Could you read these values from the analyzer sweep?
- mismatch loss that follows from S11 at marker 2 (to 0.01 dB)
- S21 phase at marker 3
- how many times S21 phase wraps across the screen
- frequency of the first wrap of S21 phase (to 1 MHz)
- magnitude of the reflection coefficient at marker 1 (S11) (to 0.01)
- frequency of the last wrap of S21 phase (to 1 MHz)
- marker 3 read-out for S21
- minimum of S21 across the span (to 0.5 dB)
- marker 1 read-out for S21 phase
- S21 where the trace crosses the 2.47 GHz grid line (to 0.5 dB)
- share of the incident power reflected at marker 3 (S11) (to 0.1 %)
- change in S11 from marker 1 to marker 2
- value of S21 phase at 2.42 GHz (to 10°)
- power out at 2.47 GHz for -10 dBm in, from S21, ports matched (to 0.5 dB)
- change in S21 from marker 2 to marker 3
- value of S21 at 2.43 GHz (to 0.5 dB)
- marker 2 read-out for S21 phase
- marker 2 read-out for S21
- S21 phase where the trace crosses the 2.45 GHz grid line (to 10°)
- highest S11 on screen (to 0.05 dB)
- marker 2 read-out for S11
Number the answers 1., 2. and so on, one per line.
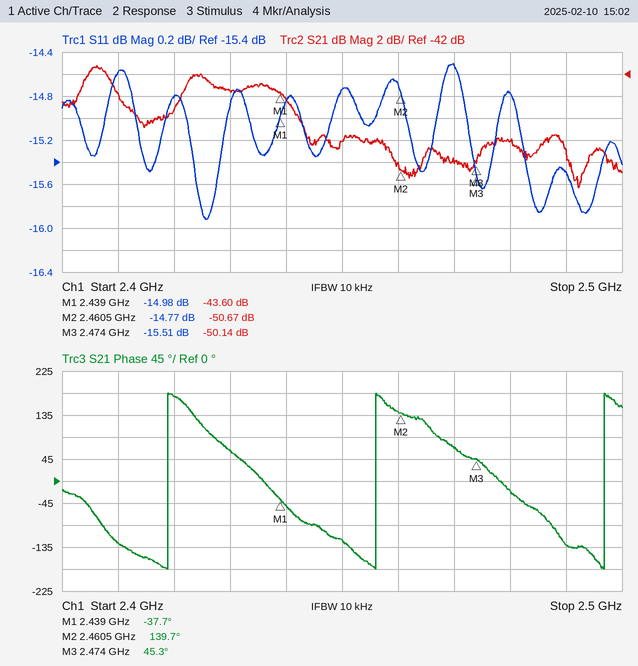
1. 0.15 dB
2. 45.3°
3. 3
4. 2.419 GHz
5. 0.18
6. 2.497 GHz
7. -50.14 dB
8. -52.5 dB
9. -37.7°
10. -50.0 dB
11. 2.8 %
12. 0.21 dB
13. 170°
14. -60.0 dBm
15. 0.53 dB
16. -43.5 dB
17. 139.7°
18. -50.67 dB
19. -120°
20. -14.50 dB
21. -14.77 dB
